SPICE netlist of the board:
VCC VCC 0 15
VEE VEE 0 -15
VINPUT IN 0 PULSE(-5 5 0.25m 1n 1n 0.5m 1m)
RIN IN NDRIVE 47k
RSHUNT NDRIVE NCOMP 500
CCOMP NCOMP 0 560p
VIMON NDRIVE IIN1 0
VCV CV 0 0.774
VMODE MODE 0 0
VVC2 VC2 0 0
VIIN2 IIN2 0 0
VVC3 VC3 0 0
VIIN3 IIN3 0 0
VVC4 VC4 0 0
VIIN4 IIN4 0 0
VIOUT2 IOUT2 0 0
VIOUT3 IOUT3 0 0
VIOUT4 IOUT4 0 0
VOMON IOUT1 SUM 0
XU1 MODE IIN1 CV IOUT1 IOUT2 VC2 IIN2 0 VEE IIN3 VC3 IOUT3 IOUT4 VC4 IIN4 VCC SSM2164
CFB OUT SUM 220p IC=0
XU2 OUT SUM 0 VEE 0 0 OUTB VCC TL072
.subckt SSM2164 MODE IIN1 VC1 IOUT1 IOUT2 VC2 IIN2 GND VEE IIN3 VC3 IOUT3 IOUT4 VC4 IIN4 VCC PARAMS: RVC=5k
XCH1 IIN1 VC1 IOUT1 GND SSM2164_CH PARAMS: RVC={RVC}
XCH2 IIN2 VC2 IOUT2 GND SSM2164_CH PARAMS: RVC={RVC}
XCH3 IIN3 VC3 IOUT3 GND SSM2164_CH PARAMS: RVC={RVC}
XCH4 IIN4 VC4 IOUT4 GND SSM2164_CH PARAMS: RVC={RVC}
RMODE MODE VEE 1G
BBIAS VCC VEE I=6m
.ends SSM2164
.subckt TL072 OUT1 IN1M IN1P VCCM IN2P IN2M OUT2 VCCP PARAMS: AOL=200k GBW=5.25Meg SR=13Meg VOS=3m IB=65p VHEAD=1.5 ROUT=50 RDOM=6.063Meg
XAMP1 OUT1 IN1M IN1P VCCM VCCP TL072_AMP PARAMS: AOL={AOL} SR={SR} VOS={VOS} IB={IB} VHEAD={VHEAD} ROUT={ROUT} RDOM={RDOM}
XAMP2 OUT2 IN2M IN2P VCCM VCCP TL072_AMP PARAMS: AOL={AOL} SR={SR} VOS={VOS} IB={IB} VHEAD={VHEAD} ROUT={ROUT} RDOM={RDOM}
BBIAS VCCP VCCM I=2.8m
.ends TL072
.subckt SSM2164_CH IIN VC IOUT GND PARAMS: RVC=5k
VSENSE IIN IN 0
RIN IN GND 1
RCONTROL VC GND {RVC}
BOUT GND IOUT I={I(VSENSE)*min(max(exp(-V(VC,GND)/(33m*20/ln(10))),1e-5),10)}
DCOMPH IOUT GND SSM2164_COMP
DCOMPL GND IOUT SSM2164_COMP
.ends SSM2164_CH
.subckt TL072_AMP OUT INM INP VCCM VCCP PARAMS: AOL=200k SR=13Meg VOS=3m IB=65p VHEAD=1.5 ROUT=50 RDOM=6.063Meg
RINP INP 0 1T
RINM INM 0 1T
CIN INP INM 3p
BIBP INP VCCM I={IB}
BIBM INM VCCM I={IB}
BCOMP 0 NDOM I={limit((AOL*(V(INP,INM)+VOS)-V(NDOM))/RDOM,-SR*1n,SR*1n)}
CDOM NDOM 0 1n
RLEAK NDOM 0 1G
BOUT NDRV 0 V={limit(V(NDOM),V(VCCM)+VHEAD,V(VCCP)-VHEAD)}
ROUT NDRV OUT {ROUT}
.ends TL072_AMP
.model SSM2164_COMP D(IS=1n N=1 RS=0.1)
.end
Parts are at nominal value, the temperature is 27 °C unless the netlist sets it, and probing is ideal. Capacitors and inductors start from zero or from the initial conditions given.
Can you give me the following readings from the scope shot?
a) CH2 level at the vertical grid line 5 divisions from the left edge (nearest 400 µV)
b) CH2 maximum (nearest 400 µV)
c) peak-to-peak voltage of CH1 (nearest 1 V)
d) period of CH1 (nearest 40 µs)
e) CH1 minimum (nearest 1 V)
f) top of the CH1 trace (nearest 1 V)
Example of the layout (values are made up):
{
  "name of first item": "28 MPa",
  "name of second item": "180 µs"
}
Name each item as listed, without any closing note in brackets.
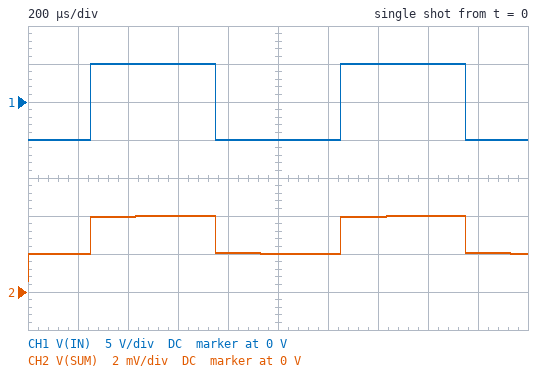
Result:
{
  "CH2 level at the vertical grid line 5 divisions from the left edge": "2.0 mV",
  "CH2 maximum": "4.0 mV",
  "peak-to-peak voltage of CH1": "10 V",
  "period of CH1": "1.00 ms",
  "CH1 minimum": "-5 V",
  "top of the CH1 trace": "5 V"
}
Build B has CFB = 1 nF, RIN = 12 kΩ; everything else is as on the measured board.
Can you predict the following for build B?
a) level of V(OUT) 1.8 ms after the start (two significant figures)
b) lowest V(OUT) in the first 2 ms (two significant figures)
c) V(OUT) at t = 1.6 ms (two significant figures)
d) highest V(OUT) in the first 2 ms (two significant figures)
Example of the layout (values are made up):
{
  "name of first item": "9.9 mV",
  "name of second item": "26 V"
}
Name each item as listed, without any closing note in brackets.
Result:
{
  "level of V(OUT) 1.8 ms after the start": "-5.6 V",
  "lowest V(OUT) in the first 2 ms": "-7.0 V",
  "V(OUT) at t = 1.6 ms": "-2.8 V",
  "highest V(OUT) in the first 2 ms": "7.0 V"
}
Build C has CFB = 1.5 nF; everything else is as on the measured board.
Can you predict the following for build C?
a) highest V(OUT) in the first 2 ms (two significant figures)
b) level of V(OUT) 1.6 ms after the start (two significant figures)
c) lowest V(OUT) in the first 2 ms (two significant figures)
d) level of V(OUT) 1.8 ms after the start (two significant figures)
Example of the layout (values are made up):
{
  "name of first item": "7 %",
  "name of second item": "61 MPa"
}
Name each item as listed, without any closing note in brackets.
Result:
{
  "highest V(OUT) in the first 2 ms": "1.2 V",
  "level of V(OUT) 1.6 ms after the start": "-470 mV",
  "lowest V(OUT) in the first 2 ms": "-1.2 V",
  "level of V(OUT) 1.8 ms after the start": "-950 mV"
}
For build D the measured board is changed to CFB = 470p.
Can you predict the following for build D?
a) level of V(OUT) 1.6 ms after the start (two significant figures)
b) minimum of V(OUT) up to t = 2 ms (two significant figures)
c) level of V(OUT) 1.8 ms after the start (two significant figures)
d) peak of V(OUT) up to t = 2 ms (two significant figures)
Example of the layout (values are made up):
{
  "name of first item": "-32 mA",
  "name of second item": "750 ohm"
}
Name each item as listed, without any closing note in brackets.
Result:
{
  "level of V(OUT) 1.6 ms after the start": "-1.5 V",
  "minimum of V(OUT) up to t = 2 ms": "-3.8 V",
  "level of V(OUT) 1.8 ms after the start": "-3.0 V",
  "peak of V(OUT) up to t = 2 ms": "3.8 V"
}
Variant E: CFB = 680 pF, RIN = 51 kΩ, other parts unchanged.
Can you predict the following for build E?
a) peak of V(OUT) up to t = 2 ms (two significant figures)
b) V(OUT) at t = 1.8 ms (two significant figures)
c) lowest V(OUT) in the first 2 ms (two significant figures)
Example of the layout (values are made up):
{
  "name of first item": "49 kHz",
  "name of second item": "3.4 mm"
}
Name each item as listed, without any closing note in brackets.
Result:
{
  "peak of V(OUT) up to t = 2 ms": "2.4 V",
  "V(OUT) at t = 1.8 ms": "-1.9 V",
  "lowest V(OUT) in the first 2 ms": "-2.4 V"
}
